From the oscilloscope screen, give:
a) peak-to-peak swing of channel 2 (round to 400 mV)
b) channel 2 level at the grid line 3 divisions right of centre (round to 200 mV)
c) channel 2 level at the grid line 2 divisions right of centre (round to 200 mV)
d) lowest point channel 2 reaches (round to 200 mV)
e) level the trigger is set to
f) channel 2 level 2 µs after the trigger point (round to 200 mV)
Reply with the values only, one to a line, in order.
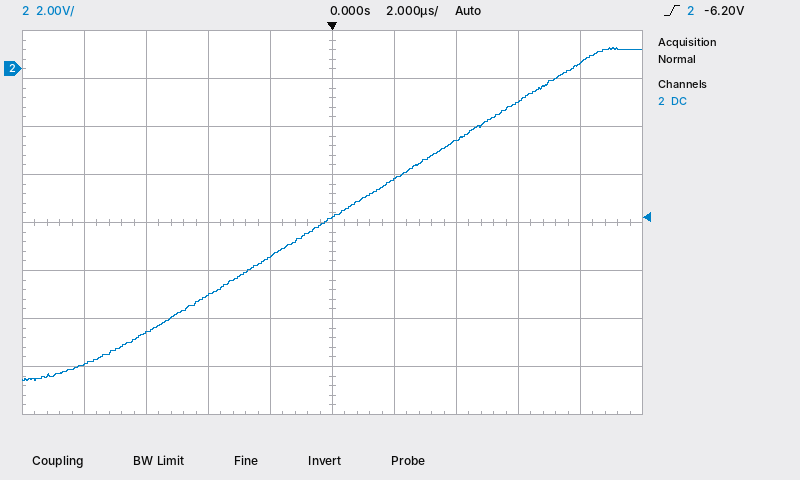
14.0 V
-1.4 V
-3.0 V
-13.0 V
-6.20 V
-4.6 V
